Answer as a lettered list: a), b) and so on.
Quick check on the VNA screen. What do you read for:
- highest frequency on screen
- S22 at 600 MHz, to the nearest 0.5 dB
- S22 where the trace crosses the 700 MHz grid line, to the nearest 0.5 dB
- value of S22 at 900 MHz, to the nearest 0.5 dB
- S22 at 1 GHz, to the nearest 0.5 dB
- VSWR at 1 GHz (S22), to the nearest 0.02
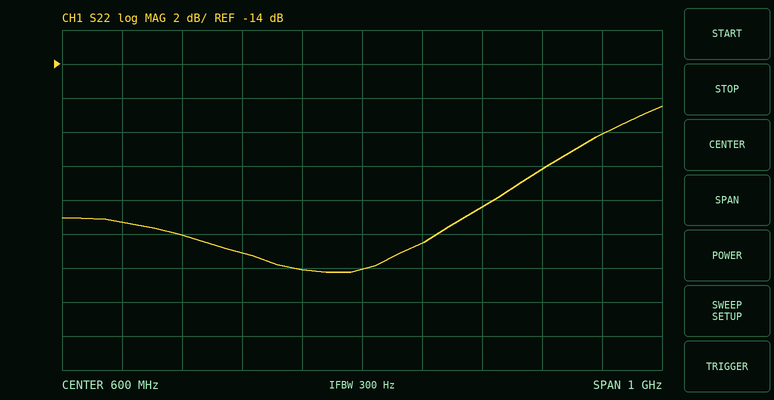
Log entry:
a) 1.1 GHz
b) -26.0 dB
c) -24.5 dB
d) -20.0 dB
e) -18.0 dB
f) 1.28
